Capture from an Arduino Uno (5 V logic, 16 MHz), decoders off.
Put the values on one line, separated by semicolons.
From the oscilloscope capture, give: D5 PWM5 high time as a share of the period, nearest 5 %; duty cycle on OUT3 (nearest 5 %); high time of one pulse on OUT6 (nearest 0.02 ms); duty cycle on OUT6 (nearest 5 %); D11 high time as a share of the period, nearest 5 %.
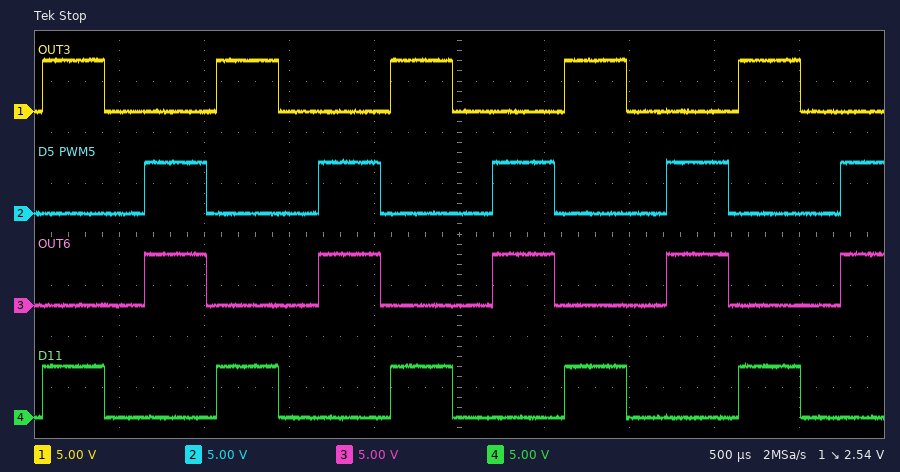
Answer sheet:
35 %; 35 %; 0.36 ms; 35 %; 35 %
